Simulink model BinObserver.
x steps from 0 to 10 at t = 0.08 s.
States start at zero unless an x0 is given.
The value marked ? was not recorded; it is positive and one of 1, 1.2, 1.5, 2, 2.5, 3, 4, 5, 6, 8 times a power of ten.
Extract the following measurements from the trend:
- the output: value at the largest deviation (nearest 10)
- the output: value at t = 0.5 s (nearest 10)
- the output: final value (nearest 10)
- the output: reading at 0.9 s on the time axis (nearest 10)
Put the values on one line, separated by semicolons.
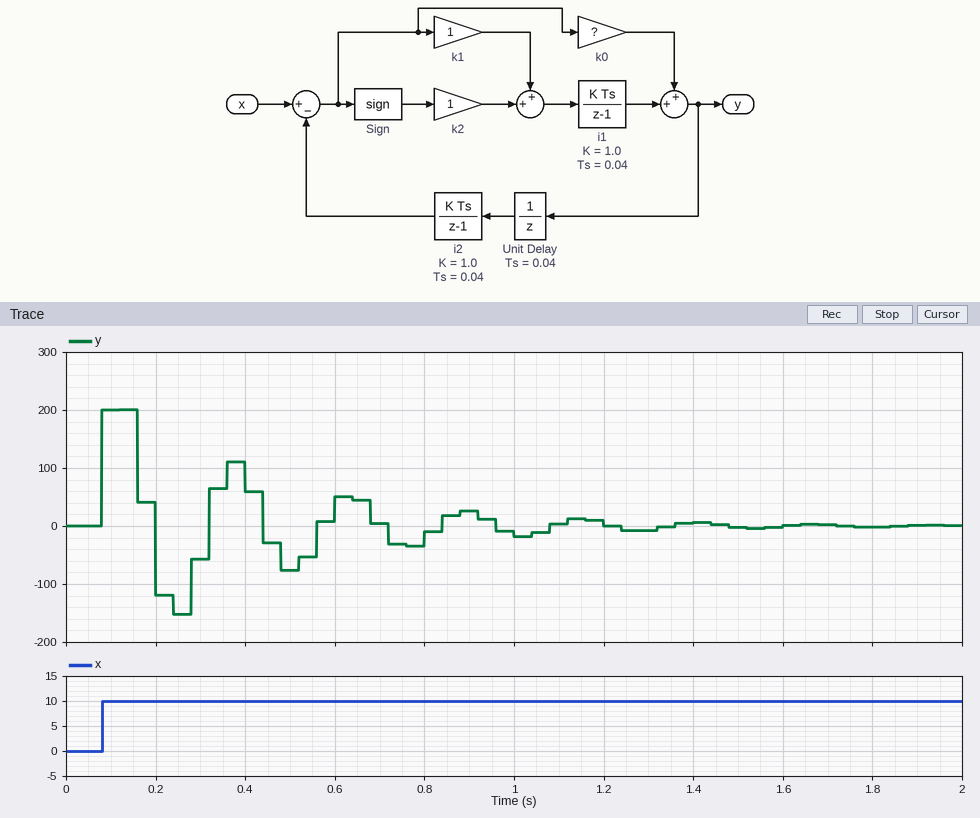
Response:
200; -80; 0; 30
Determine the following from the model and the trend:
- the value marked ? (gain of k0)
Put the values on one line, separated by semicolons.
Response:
20
